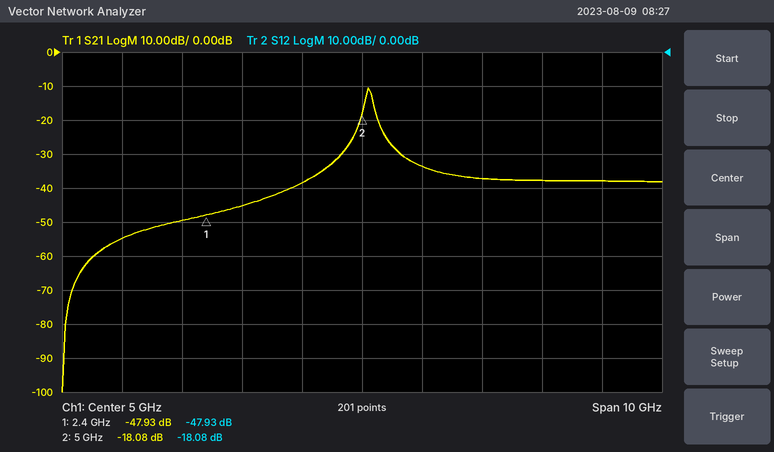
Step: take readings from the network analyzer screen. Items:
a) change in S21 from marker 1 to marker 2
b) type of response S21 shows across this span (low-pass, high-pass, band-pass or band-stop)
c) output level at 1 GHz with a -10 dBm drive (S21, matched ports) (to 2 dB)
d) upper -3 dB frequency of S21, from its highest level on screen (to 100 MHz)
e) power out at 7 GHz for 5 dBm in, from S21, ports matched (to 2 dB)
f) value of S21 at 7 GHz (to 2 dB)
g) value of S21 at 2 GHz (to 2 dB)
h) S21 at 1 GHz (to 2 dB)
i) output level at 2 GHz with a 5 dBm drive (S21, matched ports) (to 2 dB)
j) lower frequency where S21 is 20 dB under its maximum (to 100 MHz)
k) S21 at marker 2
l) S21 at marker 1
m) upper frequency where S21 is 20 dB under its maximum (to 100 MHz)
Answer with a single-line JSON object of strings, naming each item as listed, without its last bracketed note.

{"change in S21 from marker 1 to marker 2": "29.85 dB", "type of response S21 shows across this span": "band-pass", "output level at 1 GHz with a -10 dBm drive (S21, matched ports)": "-64 dBm", "upper -3 dB frequency of S21, from its highest level on screen": "5.2 GHz", "power out at 7 GHz for 5 dBm in, from S21, ports matched": "-32 dBm", "value of S21 at 7 GHz": "-38 dB", "value of S21 at 2 GHz": "-50 dB", "S21 at 1 GHz": "-54 dB", "output level at 2 GHz with a 5 dBm drive (S21, matched ports)": "-44 dBm", "lower frequency where S21 is 20 dB under its maximum": "4.6 GHz", "S21 at marker 2": "-18.08 dB", "S21 at marker 1": "-47.93 dB", "upper frequency where S21 is 20 dB under its maximum": "5.7 GHz"}
